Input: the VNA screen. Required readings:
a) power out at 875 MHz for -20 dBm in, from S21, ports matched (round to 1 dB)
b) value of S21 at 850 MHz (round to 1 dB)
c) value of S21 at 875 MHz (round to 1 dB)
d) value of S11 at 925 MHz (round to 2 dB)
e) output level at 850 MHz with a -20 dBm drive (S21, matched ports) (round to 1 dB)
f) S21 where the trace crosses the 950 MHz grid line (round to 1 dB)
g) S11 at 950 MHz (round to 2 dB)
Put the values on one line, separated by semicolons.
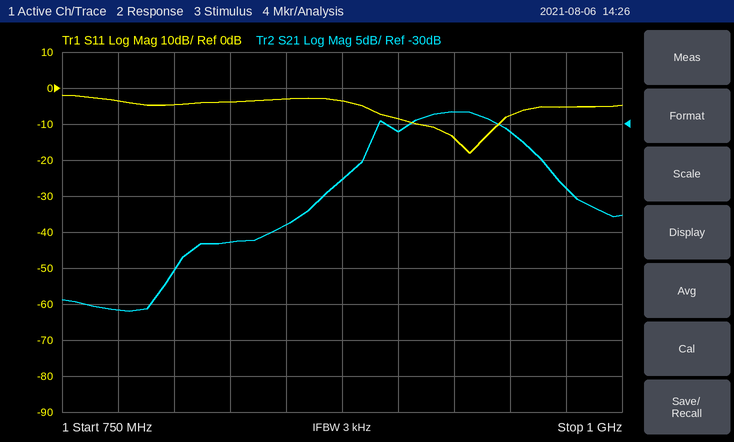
-58 dBm; -44 dB; -38 dB; -14 dB; -64 dBm; -31 dB; -8 dB
